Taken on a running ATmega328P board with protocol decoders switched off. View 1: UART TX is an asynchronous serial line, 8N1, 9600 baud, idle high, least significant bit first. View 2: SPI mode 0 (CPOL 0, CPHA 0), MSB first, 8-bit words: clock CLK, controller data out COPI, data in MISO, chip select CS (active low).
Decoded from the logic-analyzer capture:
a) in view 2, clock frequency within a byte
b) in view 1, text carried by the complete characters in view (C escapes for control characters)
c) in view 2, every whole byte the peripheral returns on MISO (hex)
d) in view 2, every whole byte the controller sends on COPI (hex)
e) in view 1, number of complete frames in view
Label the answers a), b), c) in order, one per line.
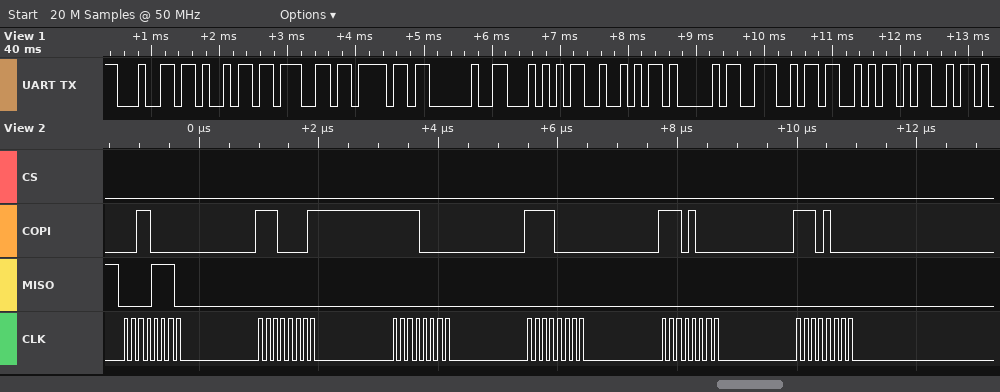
a) 8 MHz
b) "digo TRANSM"
c) 0E 00 00 00 00 00
d) 30 E1 F0 F0 E8 E8
e) 11
